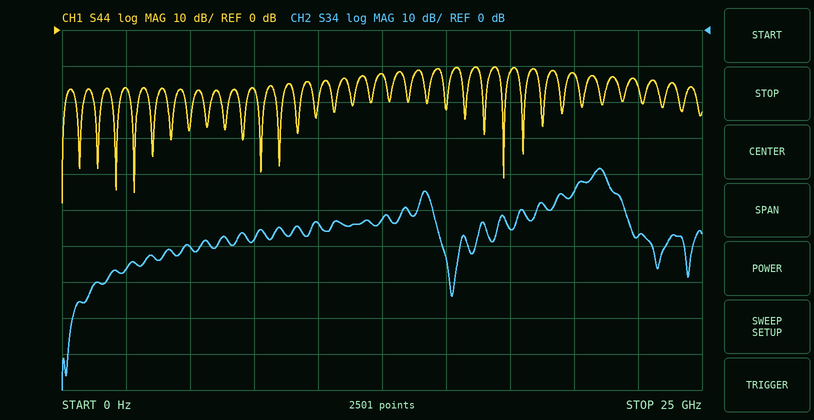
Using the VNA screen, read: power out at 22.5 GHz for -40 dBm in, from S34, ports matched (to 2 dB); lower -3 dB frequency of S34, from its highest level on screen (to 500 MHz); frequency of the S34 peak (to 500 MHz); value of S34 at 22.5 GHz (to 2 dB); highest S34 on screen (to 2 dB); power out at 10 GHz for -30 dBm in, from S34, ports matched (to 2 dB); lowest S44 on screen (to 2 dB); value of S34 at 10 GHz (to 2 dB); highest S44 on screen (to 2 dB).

-98 dBm
20.5 GHz
21.0 GHz
-58 dB
-38 dB
-84 dBm
-48 dB
-54 dB
-10 dB
